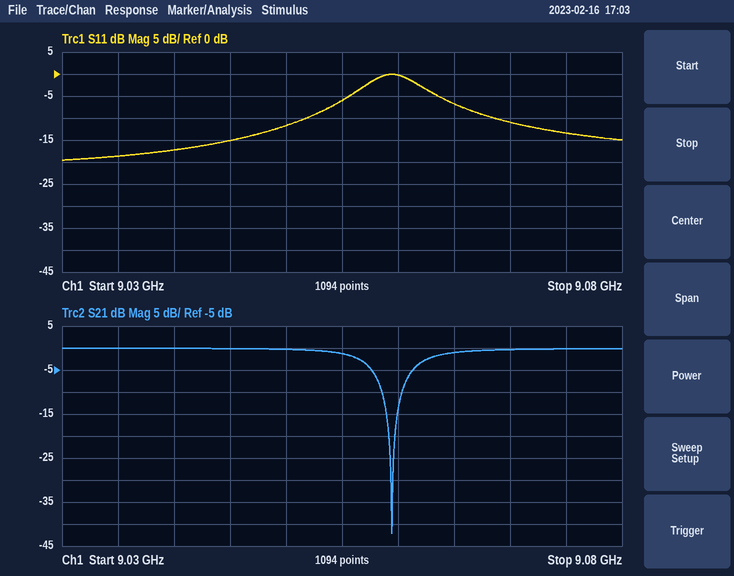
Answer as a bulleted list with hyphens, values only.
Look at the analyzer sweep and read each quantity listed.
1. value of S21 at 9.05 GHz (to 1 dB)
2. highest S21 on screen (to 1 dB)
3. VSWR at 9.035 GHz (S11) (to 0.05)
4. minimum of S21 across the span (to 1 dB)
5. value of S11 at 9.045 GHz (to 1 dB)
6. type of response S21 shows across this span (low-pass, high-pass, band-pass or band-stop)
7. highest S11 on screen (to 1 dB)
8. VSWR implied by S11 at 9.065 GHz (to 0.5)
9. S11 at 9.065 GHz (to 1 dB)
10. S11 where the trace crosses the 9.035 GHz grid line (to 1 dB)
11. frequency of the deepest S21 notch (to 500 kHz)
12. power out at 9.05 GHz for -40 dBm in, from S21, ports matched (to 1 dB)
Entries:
- 0 dB
- 0 dB
- 1.25
- -42 dB
- -15 dB
- band-stop
- 0 dB
- 2.5
- -7 dB
- -19 dB
- 9.0595 GHz
- -40 dBm
